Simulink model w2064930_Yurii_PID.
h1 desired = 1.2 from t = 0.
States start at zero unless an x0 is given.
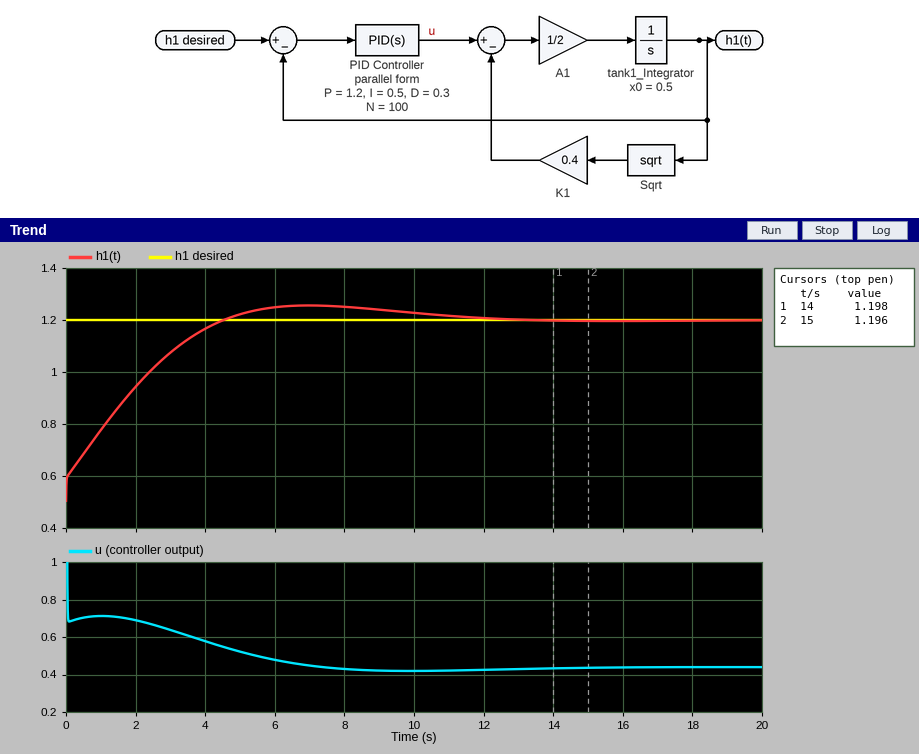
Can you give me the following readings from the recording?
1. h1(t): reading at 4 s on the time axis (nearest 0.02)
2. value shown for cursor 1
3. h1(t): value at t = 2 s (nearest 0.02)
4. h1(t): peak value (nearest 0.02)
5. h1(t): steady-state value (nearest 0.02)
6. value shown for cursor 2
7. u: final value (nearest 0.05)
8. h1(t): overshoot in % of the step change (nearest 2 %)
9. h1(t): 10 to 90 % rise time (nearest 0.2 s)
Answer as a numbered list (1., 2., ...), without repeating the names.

1. 1.16
2. 1.198
3. 0.94
4. 1.26
5. 1.20
6. 1.196
7. 0.45
8. 8 %
9. 3.6 s
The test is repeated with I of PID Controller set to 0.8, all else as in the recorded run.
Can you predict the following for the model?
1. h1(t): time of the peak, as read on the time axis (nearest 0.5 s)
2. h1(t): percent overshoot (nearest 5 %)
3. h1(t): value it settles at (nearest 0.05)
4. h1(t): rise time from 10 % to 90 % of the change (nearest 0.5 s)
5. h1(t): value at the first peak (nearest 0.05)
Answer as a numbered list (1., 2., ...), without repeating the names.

1. 5.0 s
2. 15 %
3. 1.20
4. 2.5 s
5. 1.30
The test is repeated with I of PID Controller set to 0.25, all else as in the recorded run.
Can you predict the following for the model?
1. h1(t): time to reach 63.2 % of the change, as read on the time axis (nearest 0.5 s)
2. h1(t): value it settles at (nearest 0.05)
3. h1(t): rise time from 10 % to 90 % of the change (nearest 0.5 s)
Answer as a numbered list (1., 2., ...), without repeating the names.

1. 2.5 s
2. 1.20
3. 6.0 s
